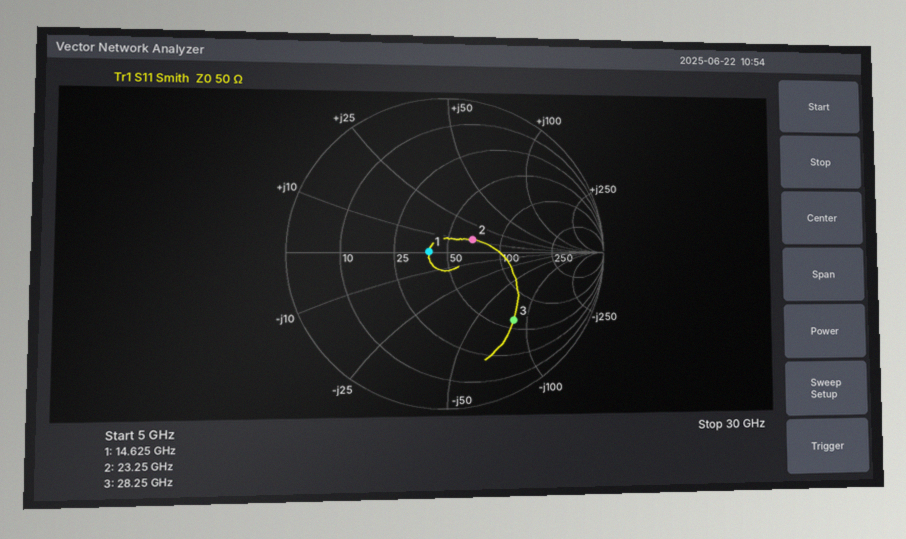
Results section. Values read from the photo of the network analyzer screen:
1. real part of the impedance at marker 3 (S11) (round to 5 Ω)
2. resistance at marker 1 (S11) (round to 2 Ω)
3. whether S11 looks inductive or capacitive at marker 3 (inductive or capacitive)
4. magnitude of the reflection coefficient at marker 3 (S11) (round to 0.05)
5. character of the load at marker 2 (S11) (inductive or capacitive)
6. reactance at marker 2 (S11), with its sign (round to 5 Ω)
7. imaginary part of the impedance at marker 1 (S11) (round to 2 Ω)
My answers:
60 Ω
40 Ω
capacitive
0.60
inductive
+10 Ω
0 Ω
